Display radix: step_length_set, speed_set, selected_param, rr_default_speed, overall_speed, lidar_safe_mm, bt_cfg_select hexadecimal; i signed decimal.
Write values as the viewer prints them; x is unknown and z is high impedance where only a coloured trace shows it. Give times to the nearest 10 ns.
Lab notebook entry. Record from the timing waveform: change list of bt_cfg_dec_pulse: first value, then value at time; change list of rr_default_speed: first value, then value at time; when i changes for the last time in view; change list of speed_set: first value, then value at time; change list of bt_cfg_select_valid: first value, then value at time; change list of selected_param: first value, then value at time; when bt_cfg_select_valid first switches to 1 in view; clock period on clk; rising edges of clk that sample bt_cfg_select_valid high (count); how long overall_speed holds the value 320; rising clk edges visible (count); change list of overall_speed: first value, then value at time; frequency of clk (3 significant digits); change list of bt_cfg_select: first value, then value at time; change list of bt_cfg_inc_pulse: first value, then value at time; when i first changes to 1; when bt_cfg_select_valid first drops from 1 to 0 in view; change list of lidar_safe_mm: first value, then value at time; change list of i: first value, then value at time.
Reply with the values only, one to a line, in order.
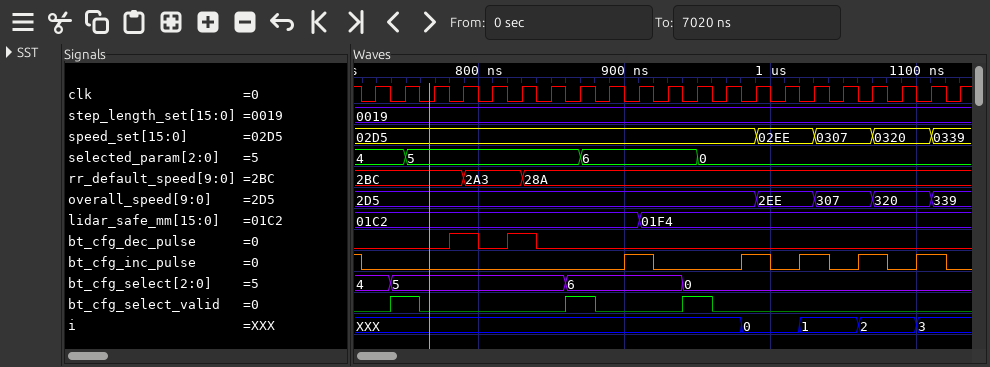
0, 1 at 780 ns, 0 at 800 ns, 1 at 820 ns, 0 at 840 ns
2BC, 2A3 at 790 ns, 28A at 830 ns
1100 ns
02D5, 02EE at 990 ns, 0307 at 1030 ns, 0320 at 1070 ns, 0339 at 1110 ns
0, 1 at 740 ns, 0 at 760 ns, 1 at 860 ns, 0 at 880 ns, 1 at 940 ns, 0 at 960 ns
4, 5 at 750 ns, 6 at 870 ns, 0 at 950 ns
740 ns
20 ns
3
40 ns
21
2D5, 2EE at 990 ns, 307 at 1030 ns, 320 at 1070 ns, 339 at 1110 ns
50.0 MHz
4, 5 at 740 ns, 6 at 860 ns, 0 at 940 ns
1, 0 at 720 ns, 1 at 900 ns, 0 at 920 ns, 1 at 980 ns, 0 at 1000 ns, 1 at 1020 ns, 0 at 1040 ns, 1 at 1060 ns, 0 at 1080 ns, 1 at 1100 ns, 0 at 1120 ns
1020 ns
760 ns
01C2, 01F4 at 910 ns
XXX, 0 at 980 ns, 1 at 1020 ns, 2 at 1060 ns, 3 at 1100 ns
